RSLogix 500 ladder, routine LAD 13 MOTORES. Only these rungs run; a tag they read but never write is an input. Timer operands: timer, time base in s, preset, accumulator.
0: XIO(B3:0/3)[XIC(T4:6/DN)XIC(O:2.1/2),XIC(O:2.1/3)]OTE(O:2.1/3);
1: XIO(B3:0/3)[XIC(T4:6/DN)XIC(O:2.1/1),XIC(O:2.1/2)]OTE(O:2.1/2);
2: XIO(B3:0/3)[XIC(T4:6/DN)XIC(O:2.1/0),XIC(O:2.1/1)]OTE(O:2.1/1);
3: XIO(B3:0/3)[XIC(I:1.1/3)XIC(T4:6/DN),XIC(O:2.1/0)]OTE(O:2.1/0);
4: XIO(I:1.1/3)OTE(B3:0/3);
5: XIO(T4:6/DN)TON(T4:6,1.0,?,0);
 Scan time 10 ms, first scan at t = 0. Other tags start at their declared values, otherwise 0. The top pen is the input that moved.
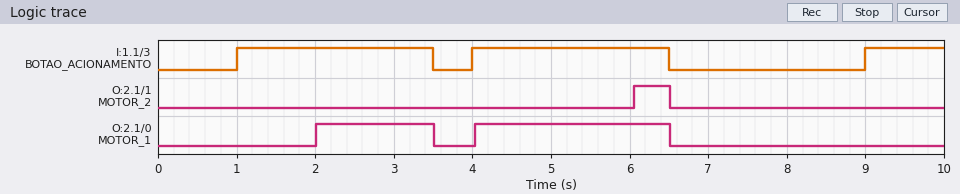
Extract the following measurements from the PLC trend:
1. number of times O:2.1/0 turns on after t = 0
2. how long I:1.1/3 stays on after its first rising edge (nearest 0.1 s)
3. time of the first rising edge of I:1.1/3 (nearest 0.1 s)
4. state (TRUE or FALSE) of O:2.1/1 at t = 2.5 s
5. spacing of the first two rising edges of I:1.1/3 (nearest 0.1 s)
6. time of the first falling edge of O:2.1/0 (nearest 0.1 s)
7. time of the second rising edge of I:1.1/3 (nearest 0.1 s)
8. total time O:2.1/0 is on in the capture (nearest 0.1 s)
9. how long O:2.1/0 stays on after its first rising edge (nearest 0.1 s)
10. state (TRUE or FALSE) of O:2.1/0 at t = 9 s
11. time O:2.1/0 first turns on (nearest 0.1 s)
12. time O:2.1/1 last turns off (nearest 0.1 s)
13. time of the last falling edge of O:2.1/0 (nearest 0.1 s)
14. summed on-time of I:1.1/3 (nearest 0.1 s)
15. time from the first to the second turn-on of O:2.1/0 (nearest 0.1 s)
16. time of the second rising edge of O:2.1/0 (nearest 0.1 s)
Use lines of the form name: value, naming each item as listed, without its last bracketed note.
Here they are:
number of times O:2.1/0 turns on after t = 0: 2
how long I:1.1/3 stays on after its first rising edge: 2.5 s
time of the first rising edge of I:1.1/3: 1.0 s
state (TRUE or FALSE) of O:2.1/1 at t = 2.5 s: FALSE
spacing of the first two rising edges of I:1.1/3: 3.0 s
time of the first falling edge of O:2.1/0: 3.5 s
time of the second rising edge of I:1.1/3: 4.0 s
total time O:2.1/0 is on in the capture: 4.0 s
how long O:2.1/0 stays on after its first rising edge: 1.5 s
state (TRUE or FALSE) of O:2.1/0 at t = 9 s: FALSE
time O:2.1/0 first turns on: 2.0 s
time O:2.1/1 last turns off: 6.5 s
time of the last falling edge of O:2.1/0: 6.5 s
summed on-time of I:1.1/3: 6.0 s
time from the first to the second turn-on of O:2.1/0: 2.0 s
time of the second rising edge of O:2.1/0: 4.0 s
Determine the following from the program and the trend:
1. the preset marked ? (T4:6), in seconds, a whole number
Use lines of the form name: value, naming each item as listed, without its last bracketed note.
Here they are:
the preset marked ? (T4:6), in seconds, a whole number: 2 s
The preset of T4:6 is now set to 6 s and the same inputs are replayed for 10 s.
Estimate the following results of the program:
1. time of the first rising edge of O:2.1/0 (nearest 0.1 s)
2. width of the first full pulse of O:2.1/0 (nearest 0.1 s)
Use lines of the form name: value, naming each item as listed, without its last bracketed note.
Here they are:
time of the first rising edge of O:2.1/0: 6.0 s
width of the first full pulse of O:2.1/0: 0.5 s
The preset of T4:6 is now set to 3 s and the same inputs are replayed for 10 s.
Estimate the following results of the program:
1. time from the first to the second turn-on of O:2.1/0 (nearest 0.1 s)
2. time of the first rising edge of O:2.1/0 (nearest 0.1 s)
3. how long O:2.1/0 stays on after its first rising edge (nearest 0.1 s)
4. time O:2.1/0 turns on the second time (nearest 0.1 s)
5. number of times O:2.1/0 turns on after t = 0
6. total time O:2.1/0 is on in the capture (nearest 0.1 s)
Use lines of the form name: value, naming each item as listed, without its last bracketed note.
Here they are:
time from the first to the second turn-on of O:2.1/0: 3.0 s
time of the first rising edge of O:2.1/0: 3.0 s
how long O:2.1/0 stays on after its first rising edge: 0.5 s
time O:2.1/0 turns on the second time: 6.0 s
number of times O:2.1/0 turns on after t = 0: 3
total time O:2.1/0 is on in the capture: 1.9 s
